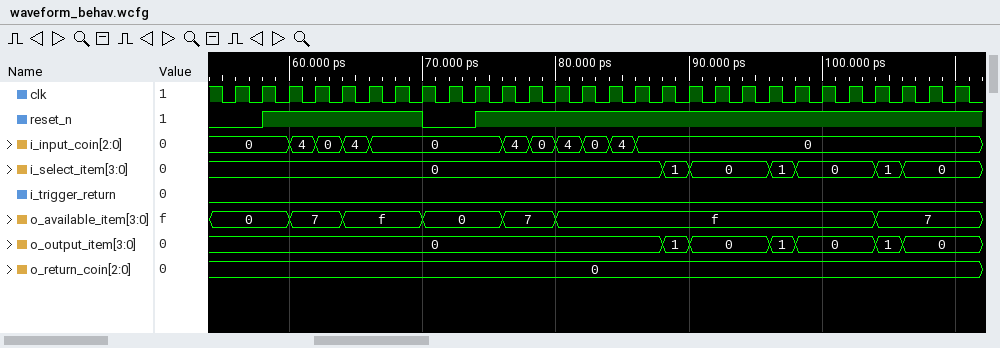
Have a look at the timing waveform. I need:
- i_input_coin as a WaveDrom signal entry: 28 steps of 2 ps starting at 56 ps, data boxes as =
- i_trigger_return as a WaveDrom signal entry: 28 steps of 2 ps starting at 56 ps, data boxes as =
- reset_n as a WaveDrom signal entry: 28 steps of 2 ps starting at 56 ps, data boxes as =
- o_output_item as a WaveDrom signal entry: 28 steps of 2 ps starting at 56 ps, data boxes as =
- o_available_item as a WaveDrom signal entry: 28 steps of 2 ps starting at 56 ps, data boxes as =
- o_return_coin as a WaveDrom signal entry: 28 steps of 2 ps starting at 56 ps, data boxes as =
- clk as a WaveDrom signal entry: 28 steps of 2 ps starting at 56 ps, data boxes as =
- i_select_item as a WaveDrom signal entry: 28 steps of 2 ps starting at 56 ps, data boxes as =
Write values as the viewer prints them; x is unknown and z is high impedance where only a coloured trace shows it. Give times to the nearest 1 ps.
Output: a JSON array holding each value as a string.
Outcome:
["{name: 'i_input_coin', wave: '=.====....======............', data: '0 4 0 4 0 4 0 4 0 4 0'}", "{name: 'i_trigger_return', wave: '0...........................'}", "{name: 'reset_n', wave: '01.....0.1..................'}", "{name: 'o_output_item', wave: '=...............==..==..==..', data: '0 1 0 1 0 1 0'}", "{name: 'o_available_item', wave: '=.=.=..=..=.=...........=...', data: '0 7 f 0 7 f 7'}", "{name: 'o_return_coin', wave: '=...........................', data: '0'}", "{name: 'clk', wave: 'p...........................'}", "{name: 'i_select_item', wave: '=...............==..==..==..', data: '0 1 0 1 0 1 0'}"]
